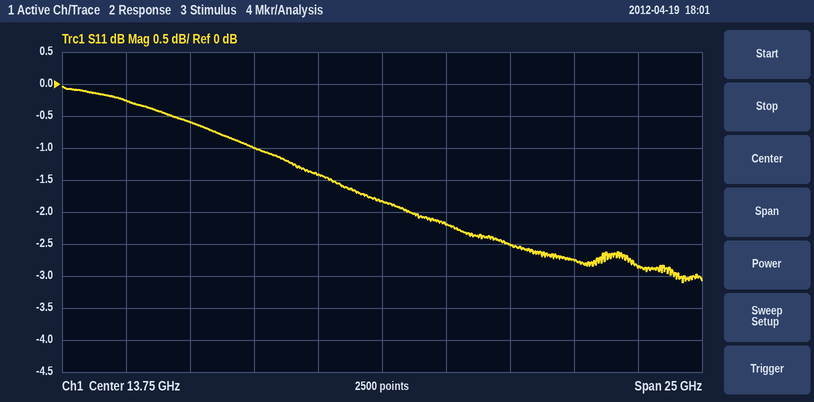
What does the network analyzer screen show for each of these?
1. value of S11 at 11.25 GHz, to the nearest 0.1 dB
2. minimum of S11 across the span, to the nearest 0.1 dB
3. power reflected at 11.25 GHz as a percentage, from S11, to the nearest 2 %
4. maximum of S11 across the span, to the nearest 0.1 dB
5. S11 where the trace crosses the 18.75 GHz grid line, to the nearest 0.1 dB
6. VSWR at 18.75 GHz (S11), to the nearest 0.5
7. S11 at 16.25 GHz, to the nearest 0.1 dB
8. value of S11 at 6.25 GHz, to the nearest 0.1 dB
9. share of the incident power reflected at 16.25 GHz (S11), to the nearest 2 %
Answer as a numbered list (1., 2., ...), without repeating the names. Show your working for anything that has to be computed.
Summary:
1. -1.4 dB
2. -3.1 dB
3. 10^(-1.4/10) ≈ 72 %
4. 0.0 dB
5. -2.5 dB
6. |Γ| = 10^(-2.5/20) = 0.7499; VSWR = (1 + 0.7499)/(1 − 0.7499) ≈ 7.0
7. -2.2 dB
8. -0.6 dB
9. 10^(-2.2/10) ≈ 60 %
